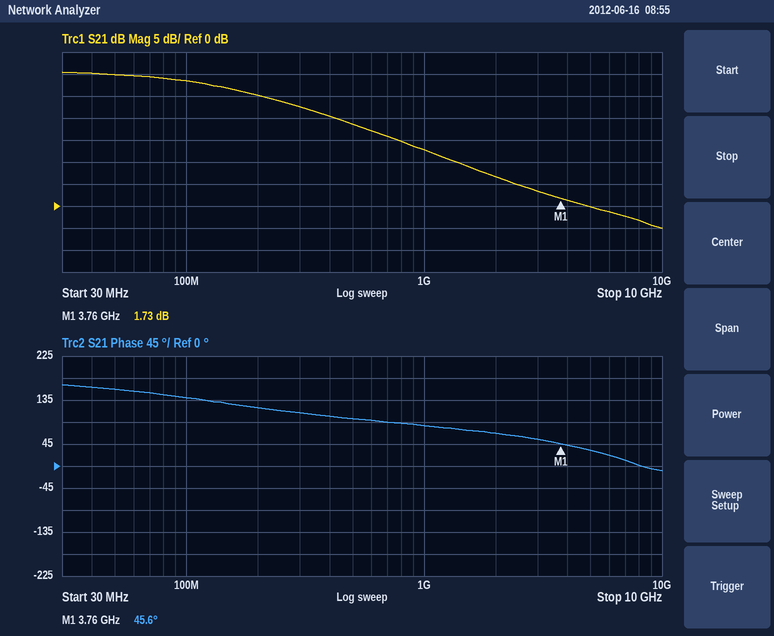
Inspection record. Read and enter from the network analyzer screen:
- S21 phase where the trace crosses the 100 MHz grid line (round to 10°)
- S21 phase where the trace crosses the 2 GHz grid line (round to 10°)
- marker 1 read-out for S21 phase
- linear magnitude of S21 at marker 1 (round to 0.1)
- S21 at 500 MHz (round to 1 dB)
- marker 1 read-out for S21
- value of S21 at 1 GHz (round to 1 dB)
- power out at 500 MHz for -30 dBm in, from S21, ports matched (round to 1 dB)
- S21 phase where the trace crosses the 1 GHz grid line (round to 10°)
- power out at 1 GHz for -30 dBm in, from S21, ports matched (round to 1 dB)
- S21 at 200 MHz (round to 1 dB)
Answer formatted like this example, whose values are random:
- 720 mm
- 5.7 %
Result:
- 140°
- 70°
- 45.6°
- 1.2
- 19 dB
- 1.73 dB
- 13 dB
- -11 dBm
- 80°
- -17 dBm
- 25 dB
